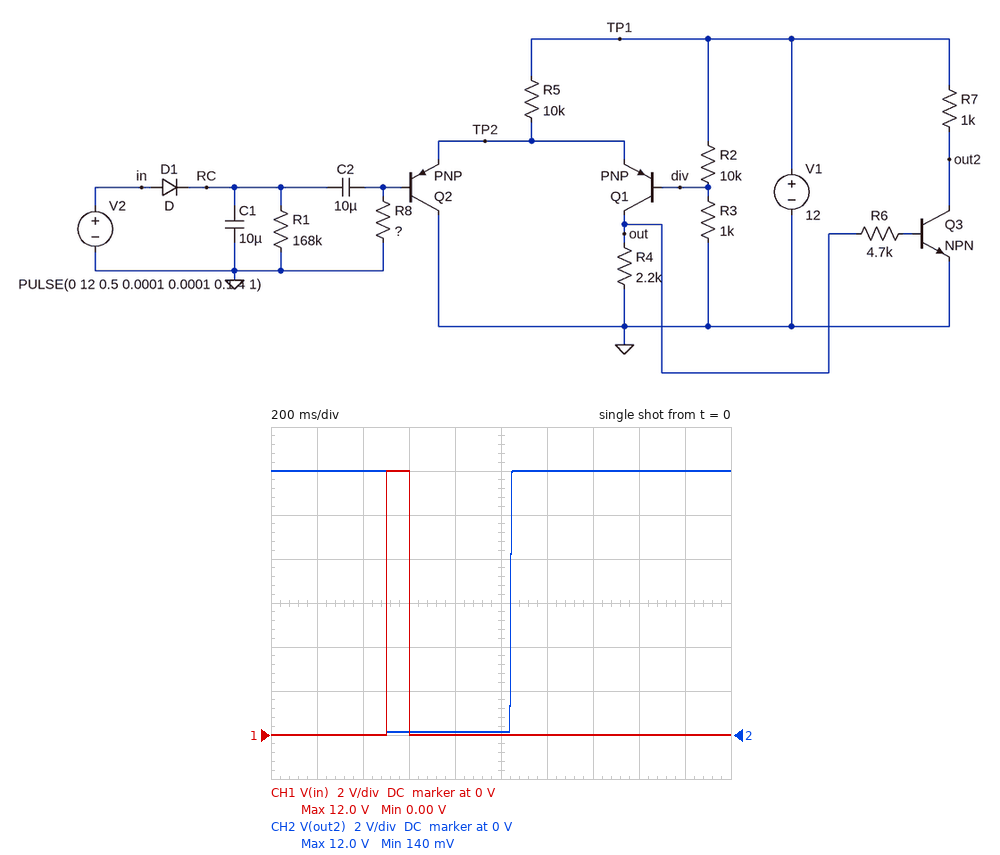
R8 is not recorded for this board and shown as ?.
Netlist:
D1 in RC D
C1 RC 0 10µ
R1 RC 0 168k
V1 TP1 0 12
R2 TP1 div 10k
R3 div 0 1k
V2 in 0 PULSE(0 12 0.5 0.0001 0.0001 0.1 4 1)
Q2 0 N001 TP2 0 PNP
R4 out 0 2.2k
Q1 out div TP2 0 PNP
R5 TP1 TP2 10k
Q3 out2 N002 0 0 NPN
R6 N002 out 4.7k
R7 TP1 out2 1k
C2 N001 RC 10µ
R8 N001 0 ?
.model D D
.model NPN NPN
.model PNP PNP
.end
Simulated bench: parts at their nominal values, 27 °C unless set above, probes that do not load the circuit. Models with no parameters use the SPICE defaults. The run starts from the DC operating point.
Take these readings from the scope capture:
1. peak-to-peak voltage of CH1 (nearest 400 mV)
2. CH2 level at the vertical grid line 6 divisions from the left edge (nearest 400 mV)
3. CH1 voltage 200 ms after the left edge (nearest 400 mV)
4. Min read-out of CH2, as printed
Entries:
12.0 V
12.0 V
0 V
140 mV
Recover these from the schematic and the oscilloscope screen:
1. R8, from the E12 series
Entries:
56 kΩ
